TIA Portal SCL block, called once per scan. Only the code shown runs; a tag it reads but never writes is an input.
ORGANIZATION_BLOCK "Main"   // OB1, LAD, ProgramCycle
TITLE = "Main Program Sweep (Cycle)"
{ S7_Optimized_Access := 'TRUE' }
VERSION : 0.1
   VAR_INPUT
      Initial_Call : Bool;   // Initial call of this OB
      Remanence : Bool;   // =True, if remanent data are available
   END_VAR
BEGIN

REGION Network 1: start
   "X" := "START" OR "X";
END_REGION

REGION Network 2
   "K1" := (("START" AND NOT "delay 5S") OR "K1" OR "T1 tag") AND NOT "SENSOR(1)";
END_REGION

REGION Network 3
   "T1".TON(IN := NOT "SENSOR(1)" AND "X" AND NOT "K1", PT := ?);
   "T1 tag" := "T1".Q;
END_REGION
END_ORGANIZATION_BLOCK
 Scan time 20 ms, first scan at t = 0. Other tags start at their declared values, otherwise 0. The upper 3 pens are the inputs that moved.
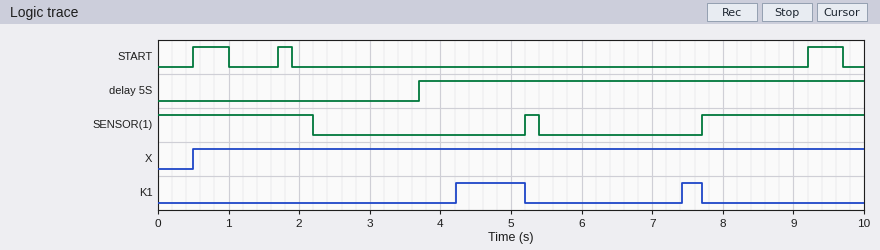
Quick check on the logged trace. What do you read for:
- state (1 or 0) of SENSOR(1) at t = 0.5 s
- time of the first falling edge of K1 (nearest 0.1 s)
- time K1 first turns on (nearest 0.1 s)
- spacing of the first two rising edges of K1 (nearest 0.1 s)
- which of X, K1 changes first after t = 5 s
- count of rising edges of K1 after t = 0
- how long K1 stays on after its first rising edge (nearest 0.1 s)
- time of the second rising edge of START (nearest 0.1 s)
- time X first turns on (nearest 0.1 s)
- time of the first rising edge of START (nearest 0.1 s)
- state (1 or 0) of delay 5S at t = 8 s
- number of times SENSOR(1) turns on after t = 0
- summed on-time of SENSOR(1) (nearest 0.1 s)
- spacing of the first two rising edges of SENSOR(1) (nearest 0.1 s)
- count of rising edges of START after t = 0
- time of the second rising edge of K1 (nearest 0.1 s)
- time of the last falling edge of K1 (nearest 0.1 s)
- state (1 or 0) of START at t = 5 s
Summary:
1
5.2 s
4.2 s
3.2 s
K1
2
1.0 s
1.7 s
0.5 s
0.5 s
1
2
4.7 s
2.5 s
3
7.4 s
7.7 s
0
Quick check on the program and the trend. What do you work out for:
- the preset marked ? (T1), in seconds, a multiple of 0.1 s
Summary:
2.0 s
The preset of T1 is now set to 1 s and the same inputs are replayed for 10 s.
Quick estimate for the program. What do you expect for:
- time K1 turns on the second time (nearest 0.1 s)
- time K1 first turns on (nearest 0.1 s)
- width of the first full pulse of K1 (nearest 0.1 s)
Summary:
6.4 s
3.2 s
2.0 s
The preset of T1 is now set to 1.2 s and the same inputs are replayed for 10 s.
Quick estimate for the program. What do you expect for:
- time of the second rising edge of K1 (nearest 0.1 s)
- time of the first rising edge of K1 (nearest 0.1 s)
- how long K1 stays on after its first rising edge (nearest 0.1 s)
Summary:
6.6 s
3.4 s
1.8 s
